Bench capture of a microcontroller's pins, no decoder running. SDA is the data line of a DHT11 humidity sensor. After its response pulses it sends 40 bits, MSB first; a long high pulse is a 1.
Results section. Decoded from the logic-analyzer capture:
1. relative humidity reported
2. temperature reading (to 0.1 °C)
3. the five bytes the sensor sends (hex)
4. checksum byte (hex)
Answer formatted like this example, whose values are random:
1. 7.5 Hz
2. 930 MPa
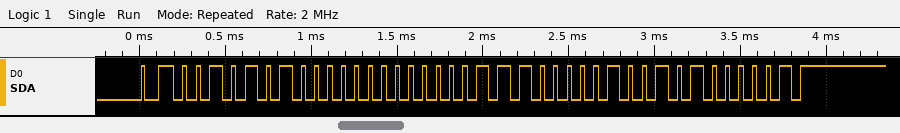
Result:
1. 42 %
2. 14.9 °C
3. 2A 00 0E 09 41
4. 0x41
